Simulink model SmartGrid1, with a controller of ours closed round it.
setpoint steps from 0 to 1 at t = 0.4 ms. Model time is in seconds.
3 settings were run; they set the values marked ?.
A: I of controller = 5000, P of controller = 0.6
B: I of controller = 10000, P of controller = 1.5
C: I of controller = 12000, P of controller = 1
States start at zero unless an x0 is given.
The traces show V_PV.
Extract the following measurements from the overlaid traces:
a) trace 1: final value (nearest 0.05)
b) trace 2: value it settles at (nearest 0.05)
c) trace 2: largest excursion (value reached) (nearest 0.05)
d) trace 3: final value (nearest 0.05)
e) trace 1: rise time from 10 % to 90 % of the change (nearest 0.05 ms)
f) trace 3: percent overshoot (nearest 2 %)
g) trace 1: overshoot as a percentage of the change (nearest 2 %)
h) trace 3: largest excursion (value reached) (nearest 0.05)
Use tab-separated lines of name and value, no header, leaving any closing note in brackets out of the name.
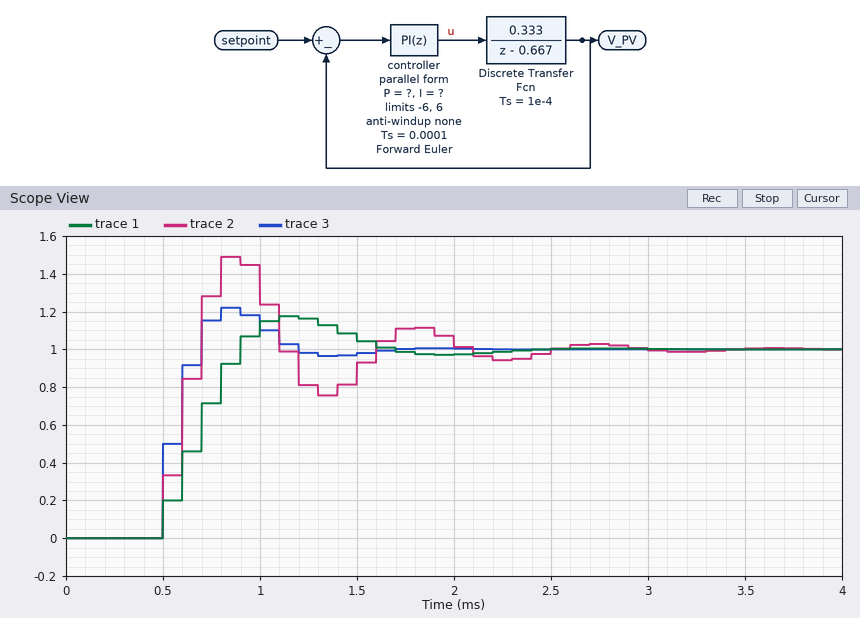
trace 1: final value	1.00
trace 2: value it settles at	1.00
trace 2: largest excursion (value reached)	1.50
trace 3: final value	1.00
trace 1: rise time from 10 % to 90 % of the change	0.30 ms
trace 3: percent overshoot	22 %
trace 1: overshoot as a percentage of the change	18 %
trace 3: largest excursion (value reached)	1.20
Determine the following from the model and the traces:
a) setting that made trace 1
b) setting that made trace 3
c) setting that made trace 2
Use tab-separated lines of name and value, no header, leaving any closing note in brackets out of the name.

setting that made trace 1	A
setting that made trace 3	B
setting that made trace 2	C
